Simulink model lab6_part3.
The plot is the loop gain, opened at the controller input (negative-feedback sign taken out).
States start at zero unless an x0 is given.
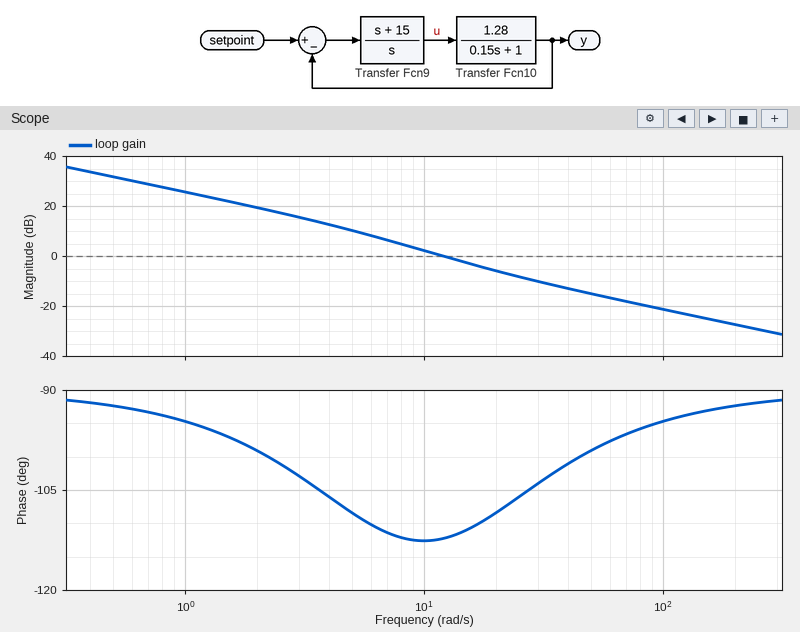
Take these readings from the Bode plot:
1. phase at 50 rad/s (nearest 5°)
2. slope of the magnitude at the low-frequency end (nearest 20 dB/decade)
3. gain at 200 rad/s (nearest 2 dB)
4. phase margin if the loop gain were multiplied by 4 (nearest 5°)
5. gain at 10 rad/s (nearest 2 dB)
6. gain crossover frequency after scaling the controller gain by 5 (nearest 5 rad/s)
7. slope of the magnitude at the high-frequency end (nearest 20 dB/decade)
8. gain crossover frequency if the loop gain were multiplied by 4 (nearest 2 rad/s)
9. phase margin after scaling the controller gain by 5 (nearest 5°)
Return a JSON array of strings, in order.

["-100°", "-20 dB/decade", "-28 dB", "80°", "2 dB", "45 rad/s", "-20 dB/decade", "36 rad/s", "80°"]
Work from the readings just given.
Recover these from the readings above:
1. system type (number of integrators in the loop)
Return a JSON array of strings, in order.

["1"]
